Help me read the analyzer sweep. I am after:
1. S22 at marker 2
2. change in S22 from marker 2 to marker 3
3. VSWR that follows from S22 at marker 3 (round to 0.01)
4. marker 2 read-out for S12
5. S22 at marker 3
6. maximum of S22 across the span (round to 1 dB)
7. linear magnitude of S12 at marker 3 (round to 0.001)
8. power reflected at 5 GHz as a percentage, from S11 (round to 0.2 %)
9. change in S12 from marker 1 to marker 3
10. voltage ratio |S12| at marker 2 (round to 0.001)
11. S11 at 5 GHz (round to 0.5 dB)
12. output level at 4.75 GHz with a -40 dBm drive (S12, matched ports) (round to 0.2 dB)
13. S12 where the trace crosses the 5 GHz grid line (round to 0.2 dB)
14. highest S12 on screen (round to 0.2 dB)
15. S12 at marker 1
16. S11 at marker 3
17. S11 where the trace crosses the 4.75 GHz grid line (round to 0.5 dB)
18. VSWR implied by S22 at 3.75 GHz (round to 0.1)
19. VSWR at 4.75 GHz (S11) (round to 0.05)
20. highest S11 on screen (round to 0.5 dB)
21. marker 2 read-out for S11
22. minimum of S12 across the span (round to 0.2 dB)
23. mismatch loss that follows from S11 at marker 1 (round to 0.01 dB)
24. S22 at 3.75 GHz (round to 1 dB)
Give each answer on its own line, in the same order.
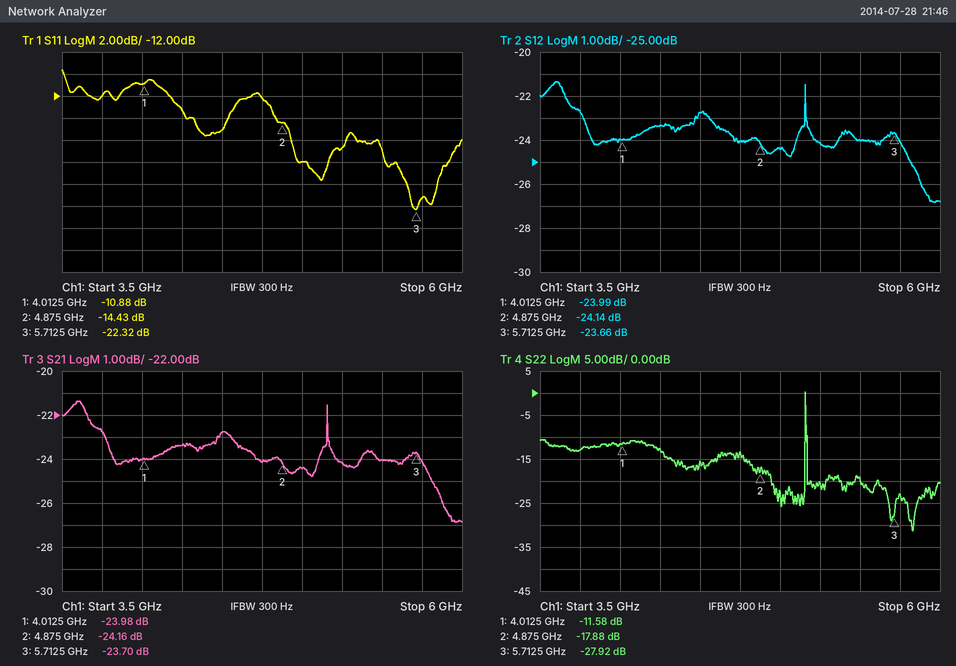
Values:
-17.88 dB
-10.04 dB
1.08
-24.14 dB
-27.92 dB
0 dB
0.066
1.6 %
0.33 dB
0.062
-18.0 dB
-64.0 dBm
-24.4 dB
-21.4 dB
-23.99 dB
-22.32 dB
-12.0 dB
1.6
1.65
-9.5 dB
-14.43 dB
-26.8 dB
0.37 dB
-13 dB
